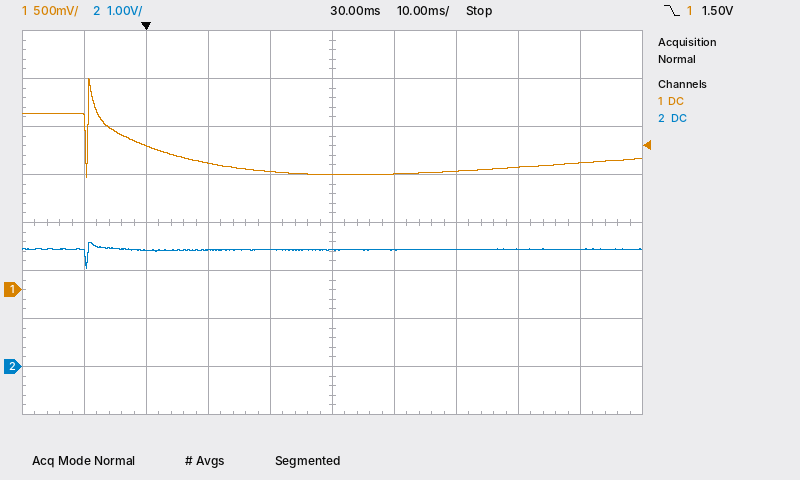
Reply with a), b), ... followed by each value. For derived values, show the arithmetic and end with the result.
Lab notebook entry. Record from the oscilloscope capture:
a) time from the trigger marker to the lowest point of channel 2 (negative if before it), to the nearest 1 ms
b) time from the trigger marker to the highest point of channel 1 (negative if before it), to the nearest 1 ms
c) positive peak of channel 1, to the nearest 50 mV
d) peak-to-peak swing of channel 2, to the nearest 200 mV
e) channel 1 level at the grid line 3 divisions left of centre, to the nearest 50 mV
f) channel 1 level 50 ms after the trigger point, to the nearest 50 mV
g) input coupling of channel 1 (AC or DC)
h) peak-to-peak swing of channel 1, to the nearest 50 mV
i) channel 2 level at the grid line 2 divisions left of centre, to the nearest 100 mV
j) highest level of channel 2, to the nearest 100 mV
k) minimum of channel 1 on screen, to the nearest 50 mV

a) -10 ms
b) -9 ms
c) 2.20 V
d) 600 mV
e) 1.50 V
f) 1.25 V
g) DC
h) 2.20 V − (1.15 V) = 1.05 V
i) 2.4 V
j) 2.6 V
k) 1.15 V
